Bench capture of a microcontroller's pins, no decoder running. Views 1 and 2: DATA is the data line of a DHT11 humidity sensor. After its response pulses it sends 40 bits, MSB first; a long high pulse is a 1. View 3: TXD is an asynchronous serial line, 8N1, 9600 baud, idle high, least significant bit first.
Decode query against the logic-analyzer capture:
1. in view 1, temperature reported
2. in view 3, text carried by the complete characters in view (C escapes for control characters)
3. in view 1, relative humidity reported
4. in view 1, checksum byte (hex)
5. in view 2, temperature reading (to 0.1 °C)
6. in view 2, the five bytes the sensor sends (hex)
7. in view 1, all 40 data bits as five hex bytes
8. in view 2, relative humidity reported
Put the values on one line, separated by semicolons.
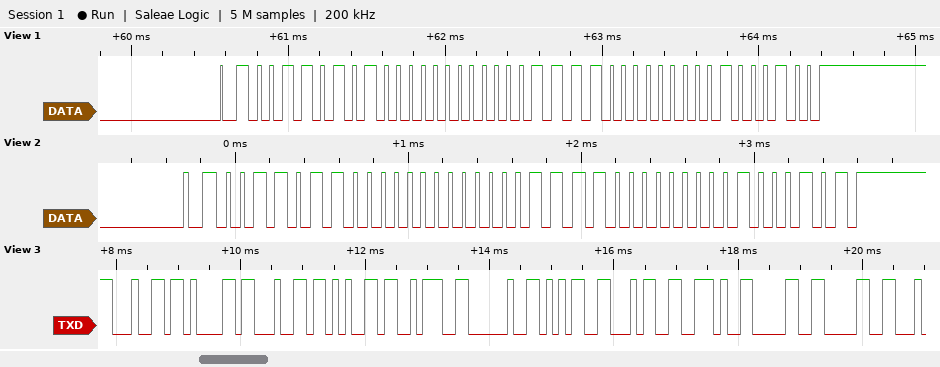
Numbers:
15.0 °C; "dade: 54.00"; 53 %; 0x44; 15.0 °C; 36 00 0F 00 45; 35 00 0F 00 44; 54 %
